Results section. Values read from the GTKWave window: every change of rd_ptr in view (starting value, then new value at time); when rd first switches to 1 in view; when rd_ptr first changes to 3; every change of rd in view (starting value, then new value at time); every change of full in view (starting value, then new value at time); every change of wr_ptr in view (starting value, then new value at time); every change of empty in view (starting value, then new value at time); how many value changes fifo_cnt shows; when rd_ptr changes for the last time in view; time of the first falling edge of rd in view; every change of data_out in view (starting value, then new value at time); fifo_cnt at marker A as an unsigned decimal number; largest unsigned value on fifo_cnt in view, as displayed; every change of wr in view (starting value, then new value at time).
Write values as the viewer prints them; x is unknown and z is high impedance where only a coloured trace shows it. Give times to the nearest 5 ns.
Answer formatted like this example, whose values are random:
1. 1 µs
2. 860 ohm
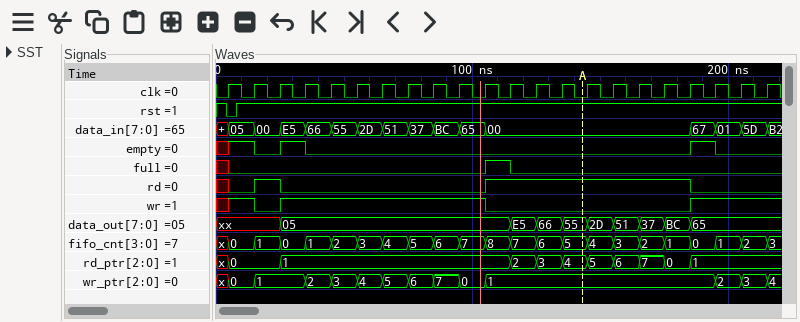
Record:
1. x, 0 at 5 ns, 1 at 25 ns, 2 at 115 ns, 3 at 125 ns, 4 at 135 ns, 5 at 145 ns, 6 at 155 ns, 7 at 165 ns, 0 at 175 ns, 1 at 185 ns
2. 15 ns
3. 125 ns
4. x, 0 at 5 ns, 1 at 15 ns, 0 at 25 ns, 1 at 105 ns, 0 at 185 ns
5. x, 0 at 5 ns, 1 at 105 ns, 0 at 115 ns
6. x, 0 at 5 ns, 1 at 15 ns, 2 at 35 ns, 3 at 45 ns, 4 at 55 ns, 5 at 65 ns, 6 at 75 ns, 7 at 85 ns, 0 at 95 ns, 1 at 105 ns, 2 at 195 ns, 3 at 205 ns, 4 at 215 ns
7. x, 1 at 5 ns, 0 at 15 ns, 1 at 25 ns, 0 at 35 ns, 1 at 185 ns, 0 at 195 ns
8. 22
9. 185 ns
10. 25 ns
11. xx, 05 at 25 ns, E5 at 115 ns, 66 at 125 ns, 55 at 135 ns, 2D at 145 ns, 51 at 155 ns, 37 at 165 ns, BC at 175 ns, 65 at 185 ns
12. 5
13. 8
14. x, 1 at 5 ns, 0 at 15 ns, 1 at 25 ns, 0 at 105 ns, 1 at 185 ns
